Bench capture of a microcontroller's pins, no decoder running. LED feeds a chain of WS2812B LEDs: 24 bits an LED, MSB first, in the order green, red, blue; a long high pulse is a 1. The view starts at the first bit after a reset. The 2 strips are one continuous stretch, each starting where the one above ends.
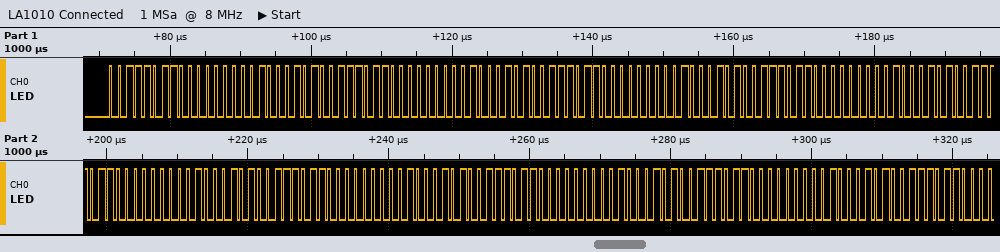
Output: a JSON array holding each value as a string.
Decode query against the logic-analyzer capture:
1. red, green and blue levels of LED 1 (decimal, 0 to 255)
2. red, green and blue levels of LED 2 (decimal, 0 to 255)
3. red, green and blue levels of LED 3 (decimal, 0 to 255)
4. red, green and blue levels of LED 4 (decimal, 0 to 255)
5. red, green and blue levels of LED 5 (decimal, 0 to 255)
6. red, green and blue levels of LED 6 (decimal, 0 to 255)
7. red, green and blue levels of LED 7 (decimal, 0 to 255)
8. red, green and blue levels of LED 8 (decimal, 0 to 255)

["0, 59, 69", "0, 59, 69", "0, 59, 69", "0, 59, 69", "0, 59, 69", "0, 59, 69", "0, 59, 69", "0, 59, 69"]
